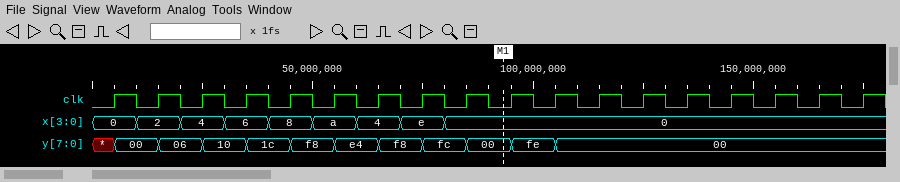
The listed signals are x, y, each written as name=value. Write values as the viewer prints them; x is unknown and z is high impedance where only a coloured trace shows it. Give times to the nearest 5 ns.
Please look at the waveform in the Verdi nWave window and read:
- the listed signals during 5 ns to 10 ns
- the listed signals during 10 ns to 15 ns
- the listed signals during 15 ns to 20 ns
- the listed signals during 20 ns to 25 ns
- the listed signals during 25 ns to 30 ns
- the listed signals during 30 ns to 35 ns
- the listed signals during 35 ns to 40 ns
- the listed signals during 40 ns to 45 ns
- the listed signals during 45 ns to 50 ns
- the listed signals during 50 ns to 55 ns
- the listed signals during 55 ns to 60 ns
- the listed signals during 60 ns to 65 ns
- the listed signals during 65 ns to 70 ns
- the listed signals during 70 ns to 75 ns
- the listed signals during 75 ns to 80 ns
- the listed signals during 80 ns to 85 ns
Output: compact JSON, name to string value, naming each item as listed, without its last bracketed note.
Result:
{"the listed signals during 5 ns to 10 ns": "x=0, y=00", "the listed signals during 10 ns to 15 ns": "x=2, y=00", "the listed signals during 15 ns to 20 ns": "x=2, y=06", "the listed signals during 20 ns to 25 ns": "x=4, y=06", "the listed signals during 25 ns to 30 ns": "x=4, y=10", "the listed signals during 30 ns to 35 ns": "x=6, y=10", "the listed signals during 35 ns to 40 ns": "x=6, y=1c", "the listed signals during 40 ns to 45 ns": "x=8, y=1c", "the listed signals during 45 ns to 50 ns": "x=8, y=f8", "the listed signals during 50 ns to 55 ns": "x=a, y=f8", "the listed signals during 55 ns to 60 ns": "x=a, y=e4", "the listed signals during 60 ns to 65 ns": "x=4, y=e4", "the listed signals during 65 ns to 70 ns": "x=4, y=f8", "the listed signals during 70 ns to 75 ns": "x=e, y=f8", "the listed signals during 75 ns to 80 ns": "x=e, y=fc", "the listed signals during 80 ns to 85 ns": "x=0, y=fc"}
